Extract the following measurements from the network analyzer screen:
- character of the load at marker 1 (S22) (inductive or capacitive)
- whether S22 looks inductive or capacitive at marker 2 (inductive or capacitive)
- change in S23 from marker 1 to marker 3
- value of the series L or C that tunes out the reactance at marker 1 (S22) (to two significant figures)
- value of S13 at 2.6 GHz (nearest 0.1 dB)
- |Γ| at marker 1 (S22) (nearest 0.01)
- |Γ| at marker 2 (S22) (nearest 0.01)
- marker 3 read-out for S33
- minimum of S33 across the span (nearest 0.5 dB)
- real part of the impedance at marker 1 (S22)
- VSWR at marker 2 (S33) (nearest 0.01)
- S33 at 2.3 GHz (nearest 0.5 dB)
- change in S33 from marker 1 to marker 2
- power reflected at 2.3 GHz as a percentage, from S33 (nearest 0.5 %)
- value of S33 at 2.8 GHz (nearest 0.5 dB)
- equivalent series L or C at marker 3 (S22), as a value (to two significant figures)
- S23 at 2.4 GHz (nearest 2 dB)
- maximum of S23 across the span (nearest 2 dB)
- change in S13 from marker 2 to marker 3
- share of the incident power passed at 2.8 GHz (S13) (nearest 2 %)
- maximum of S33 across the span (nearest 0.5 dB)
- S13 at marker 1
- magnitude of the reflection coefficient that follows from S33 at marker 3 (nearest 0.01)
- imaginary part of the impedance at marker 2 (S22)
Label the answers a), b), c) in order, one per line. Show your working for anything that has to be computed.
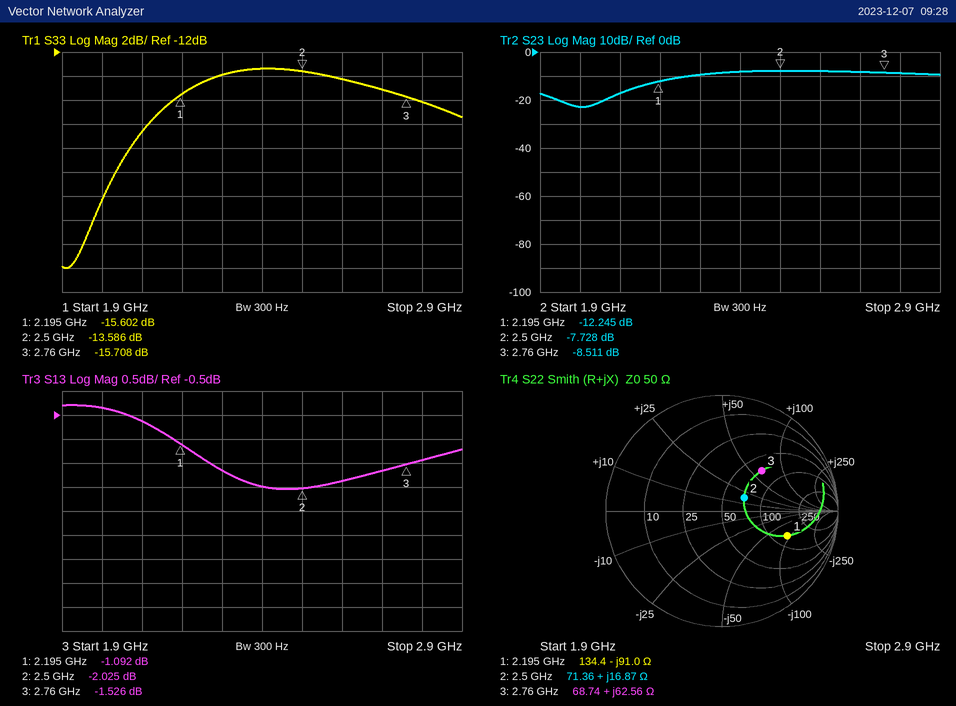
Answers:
a) capacitive
b) inductive
c) -8.511 − (-12.245) = 3.734 dB
d) L = 91 Ω/(2π × 2.195 GHz) ≈ 6.6 nH
e) -1.9 dB
f) 0.60
g) 0.22
h) -15.708 dB
i) -30.0 dB
j) 134.4 Ω
k) (1 + 0.2093)/(1 − 0.2093) ≈ 1.53
l) -14.0 dB
m) -13.586 − (-15.602) = 2.016 dB
n) 10^(-14/10) ≈ 4.0 %
o) -16.0 dB
p) L = 62.56 Ω/(2π × 2.76 GHz) ≈ 3.6 nH
q) -8 dB
r) -8 dB
s) -1.526 − (-2.025) = 0.499 dB
t) 10^(-1.4/10) ≈ 72 %
u) -13.5 dB
v) -1.092 dB
w) 10^(-15.708/20) ≈ 0.16
x) +16.87 Ω
